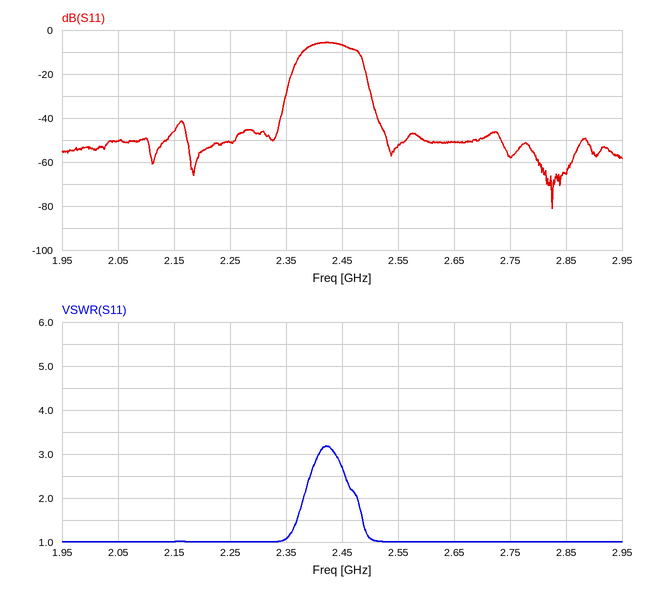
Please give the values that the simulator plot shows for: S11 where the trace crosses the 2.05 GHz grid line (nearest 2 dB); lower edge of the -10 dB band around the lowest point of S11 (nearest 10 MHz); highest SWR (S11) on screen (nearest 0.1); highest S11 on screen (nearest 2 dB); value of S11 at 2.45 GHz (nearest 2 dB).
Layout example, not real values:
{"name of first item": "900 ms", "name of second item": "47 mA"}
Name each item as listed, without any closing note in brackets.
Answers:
{"S11 where the trace crosses the 2.05 GHz grid line": "-50 dB", "lower edge of the -10 dB band around the lowest point of S11": "2.48 GHz", "highest SWR (S11) on screen": "3.2", "highest S11 on screen": "-6 dB", "value of S11 at 2.45 GHz": "-6 dB"}
